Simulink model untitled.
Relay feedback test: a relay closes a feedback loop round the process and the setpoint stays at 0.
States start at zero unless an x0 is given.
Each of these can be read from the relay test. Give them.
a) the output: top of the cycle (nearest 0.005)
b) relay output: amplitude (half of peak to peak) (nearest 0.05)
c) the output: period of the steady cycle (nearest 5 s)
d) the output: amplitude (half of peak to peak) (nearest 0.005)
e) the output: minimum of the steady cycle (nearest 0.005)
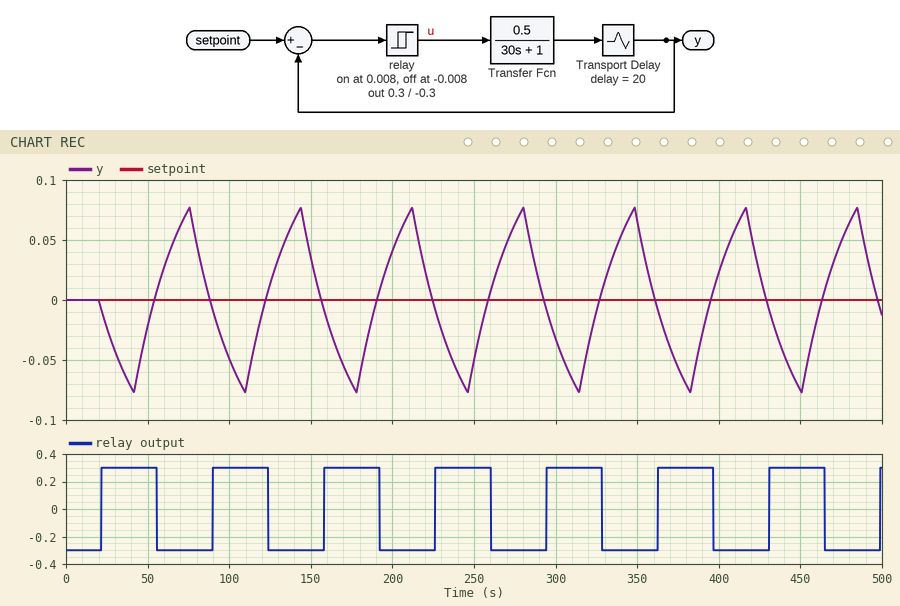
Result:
0.075
0.30
70 s
0.075
-0.075
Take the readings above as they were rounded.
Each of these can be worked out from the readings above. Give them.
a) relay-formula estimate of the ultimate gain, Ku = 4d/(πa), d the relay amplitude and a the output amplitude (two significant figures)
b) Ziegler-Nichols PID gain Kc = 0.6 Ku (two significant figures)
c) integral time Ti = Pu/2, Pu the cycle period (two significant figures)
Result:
5.1
3.1
35 s
